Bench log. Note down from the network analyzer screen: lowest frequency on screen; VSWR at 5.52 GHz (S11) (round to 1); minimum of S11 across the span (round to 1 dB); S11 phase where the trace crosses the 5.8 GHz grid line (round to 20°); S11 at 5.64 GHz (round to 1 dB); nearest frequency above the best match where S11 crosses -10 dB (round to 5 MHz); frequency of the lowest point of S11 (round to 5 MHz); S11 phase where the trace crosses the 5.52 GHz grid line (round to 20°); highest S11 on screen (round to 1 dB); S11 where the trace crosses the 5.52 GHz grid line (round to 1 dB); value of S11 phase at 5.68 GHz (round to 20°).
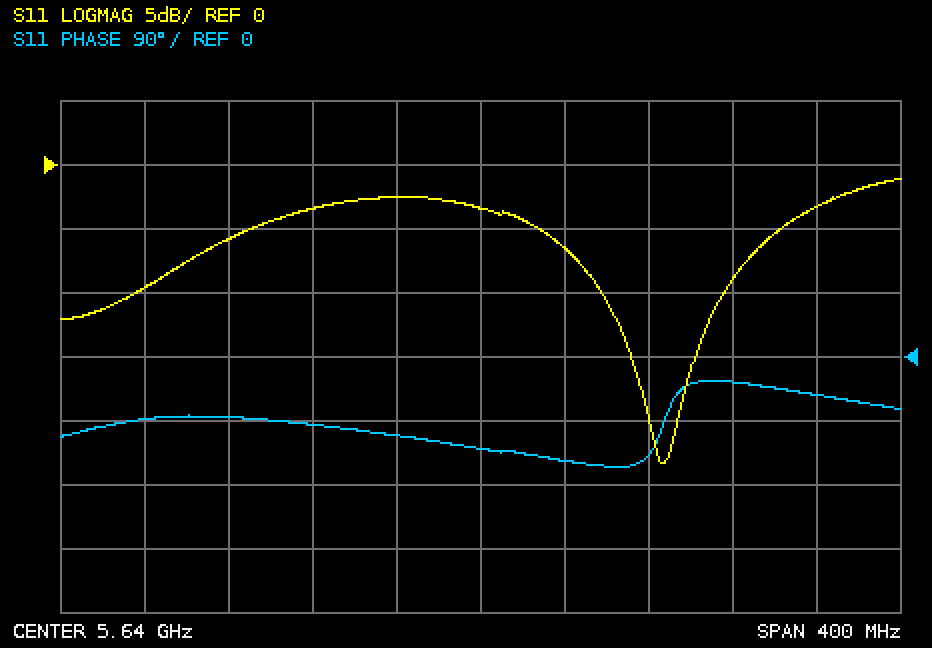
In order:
5.44 GHz
3
-23 dB
-60°
-3 dB
5.755 GHz
5.725 GHz
-80°
-1 dB
-6 dB
-140°
